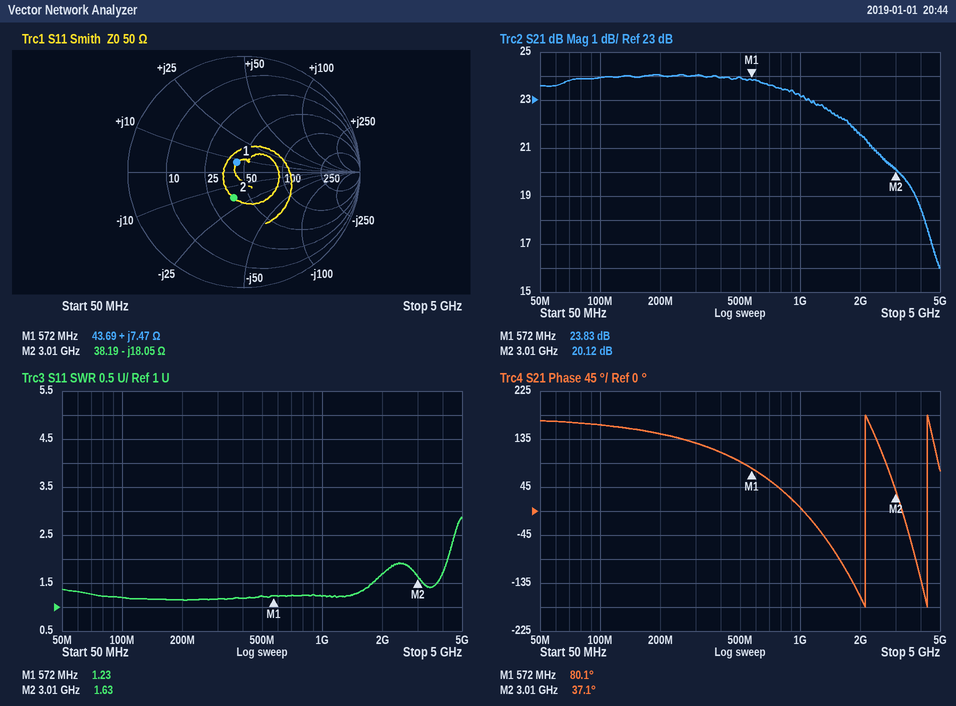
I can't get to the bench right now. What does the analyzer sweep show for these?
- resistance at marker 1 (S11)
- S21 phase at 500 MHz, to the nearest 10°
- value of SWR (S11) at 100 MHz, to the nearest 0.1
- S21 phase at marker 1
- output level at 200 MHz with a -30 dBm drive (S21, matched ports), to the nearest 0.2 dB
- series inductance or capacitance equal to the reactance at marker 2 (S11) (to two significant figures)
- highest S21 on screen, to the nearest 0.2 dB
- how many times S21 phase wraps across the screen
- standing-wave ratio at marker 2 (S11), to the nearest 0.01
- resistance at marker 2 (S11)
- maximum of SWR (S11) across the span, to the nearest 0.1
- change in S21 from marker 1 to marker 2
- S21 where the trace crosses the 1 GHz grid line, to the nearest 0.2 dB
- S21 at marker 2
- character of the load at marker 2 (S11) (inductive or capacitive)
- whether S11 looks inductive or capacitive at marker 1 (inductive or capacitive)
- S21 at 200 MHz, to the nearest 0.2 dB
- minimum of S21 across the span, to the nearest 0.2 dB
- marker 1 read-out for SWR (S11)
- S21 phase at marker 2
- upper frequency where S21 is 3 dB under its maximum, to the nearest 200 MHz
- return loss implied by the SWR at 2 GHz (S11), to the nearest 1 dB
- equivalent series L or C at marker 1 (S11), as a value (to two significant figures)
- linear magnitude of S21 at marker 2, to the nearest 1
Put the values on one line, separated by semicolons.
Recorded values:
43.69 Ω; 90°; 1.2; 80.1°; -6.0 dBm; 2.9 pF; 24.0 dB; 2; 1.63; 38.19 Ω; 2.9; -3.71 dB; 23.2 dB; 20.12 dB; capacitive; inductive; 24.0 dB; 16.0 dB; 1.23; 37.1°; 2.2 GHz; 12 dB; 2.1 nH; 10
